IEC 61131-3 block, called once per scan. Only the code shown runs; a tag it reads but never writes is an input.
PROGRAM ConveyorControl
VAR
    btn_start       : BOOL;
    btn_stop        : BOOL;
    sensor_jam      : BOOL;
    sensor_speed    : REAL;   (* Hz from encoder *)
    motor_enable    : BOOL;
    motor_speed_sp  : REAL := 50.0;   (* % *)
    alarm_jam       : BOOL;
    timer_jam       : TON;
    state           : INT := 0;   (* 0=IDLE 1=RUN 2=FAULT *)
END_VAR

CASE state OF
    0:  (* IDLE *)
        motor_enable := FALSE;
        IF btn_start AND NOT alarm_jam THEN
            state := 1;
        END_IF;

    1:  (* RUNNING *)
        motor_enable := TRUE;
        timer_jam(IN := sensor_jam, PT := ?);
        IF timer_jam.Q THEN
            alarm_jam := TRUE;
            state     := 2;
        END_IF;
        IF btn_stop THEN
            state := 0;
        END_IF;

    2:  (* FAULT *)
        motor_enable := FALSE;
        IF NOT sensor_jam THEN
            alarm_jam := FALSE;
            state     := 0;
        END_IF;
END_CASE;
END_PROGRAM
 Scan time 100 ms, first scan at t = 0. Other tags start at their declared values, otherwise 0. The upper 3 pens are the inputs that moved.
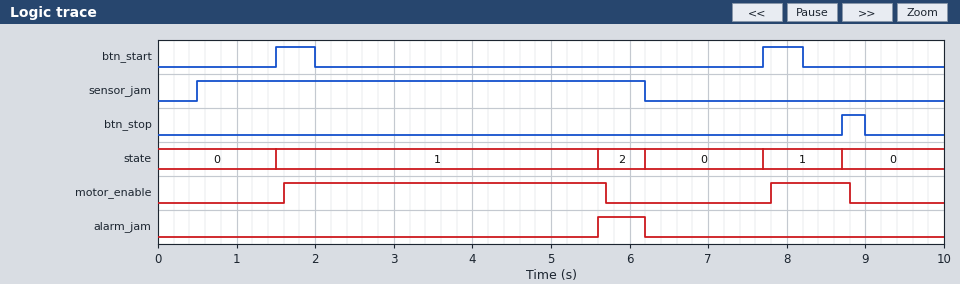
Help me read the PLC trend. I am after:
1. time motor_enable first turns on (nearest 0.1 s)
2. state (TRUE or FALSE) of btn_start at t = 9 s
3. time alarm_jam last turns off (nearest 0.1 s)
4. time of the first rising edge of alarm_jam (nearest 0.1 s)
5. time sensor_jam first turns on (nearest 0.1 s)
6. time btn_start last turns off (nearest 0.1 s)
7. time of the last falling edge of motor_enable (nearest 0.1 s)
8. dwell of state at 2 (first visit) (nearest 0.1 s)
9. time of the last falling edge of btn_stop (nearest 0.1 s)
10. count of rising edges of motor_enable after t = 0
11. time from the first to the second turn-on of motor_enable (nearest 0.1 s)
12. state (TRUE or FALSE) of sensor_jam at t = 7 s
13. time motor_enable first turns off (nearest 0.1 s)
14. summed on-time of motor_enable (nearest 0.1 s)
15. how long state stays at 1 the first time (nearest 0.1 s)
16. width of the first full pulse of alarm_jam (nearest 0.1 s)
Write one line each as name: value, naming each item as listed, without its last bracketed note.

time motor_enable first turns on: 1.6 s
state (TRUE or FALSE) of btn_start at t = 9 s: FALSE
time alarm_jam last turns off: 6.2 s
time of the first rising edge of alarm_jam: 5.6 s
time sensor_jam first turns on: 0.5 s
time btn_start last turns off: 8.2 s
time of the last falling edge of motor_enable: 8.8 s
dwell of state at 2 (first visit): 0.6 s
time of the last falling edge of btn_stop: 9.0 s
count of rising edges of motor_enable after t = 0: 2
time from the first to the second turn-on of motor_enable: 6.2 s
state (TRUE or FALSE) of sensor_jam at t = 7 s: FALSE
time motor_enable first turns off: 5.7 s
summed on-time of motor_enable: 5.1 s
how long state stays at 1 the first time: 4.1 s
width of the first full pulse of alarm_jam: 0.6 s
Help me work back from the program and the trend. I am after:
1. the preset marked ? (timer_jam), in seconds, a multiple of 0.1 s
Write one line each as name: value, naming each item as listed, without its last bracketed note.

the preset marked ? (timer_jam), in seconds, a multiple of 0.1 s: 4.0 s
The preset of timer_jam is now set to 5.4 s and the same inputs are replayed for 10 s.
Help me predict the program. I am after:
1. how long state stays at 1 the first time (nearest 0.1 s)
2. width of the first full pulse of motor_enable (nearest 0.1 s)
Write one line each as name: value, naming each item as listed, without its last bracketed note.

how long state stays at 1 the first time: 7.2 s
width of the first full pulse of motor_enable: 7.2 s
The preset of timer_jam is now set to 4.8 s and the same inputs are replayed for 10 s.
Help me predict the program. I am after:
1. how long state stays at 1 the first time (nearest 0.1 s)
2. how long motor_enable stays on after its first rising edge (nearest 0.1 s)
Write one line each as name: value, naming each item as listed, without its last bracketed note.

how long state stays at 1 the first time: 7.2 s
how long motor_enable stays on after its first rising edge: 7.2 s
